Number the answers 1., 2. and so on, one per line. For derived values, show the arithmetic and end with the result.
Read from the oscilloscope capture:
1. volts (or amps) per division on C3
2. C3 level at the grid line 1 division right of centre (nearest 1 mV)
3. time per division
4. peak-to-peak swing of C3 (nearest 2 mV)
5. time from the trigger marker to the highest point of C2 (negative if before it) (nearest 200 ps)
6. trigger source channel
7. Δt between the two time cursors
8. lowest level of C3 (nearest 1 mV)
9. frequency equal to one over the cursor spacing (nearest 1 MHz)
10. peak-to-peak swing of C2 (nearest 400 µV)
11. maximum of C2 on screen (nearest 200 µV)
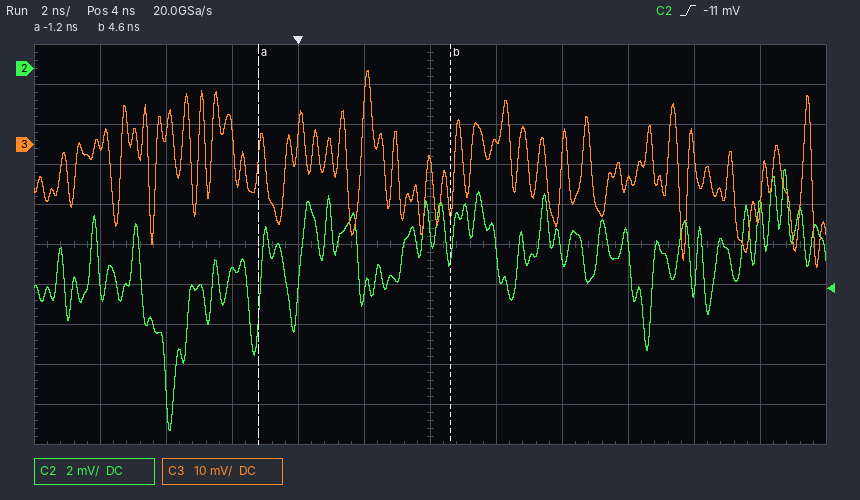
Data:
1. 10 mV
2. 1 mV
3. 2 ns
4. 50 mV
5. +14.8 ns
6. C2
7. 4.6 ns − (-1.2 ns) = 5.8 ns
8. -31 mV
9. 1 / 5.8 ns ≈ 172 MHz
10. 13.2 mV
11. -5.0 mV
